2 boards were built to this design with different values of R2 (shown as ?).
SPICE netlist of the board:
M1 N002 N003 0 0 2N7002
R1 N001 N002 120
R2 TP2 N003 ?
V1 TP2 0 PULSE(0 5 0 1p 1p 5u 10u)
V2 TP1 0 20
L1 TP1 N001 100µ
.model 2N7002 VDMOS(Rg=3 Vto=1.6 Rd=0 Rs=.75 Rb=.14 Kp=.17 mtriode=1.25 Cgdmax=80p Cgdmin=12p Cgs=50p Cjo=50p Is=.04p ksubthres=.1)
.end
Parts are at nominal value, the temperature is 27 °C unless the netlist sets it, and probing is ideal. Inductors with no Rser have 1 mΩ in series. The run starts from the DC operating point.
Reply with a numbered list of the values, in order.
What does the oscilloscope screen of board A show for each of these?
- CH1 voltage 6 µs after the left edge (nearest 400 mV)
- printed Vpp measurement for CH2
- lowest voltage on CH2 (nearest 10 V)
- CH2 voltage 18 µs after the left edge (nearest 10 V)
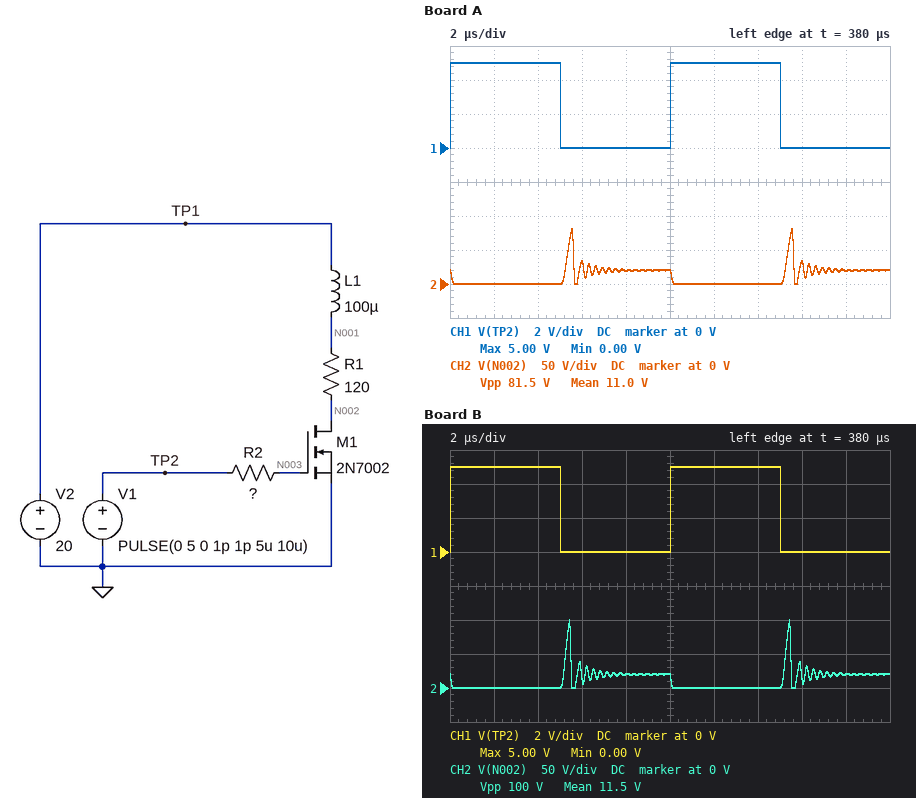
1. 0 V
2. 81.5 V
3. 0 V
4. 20 V
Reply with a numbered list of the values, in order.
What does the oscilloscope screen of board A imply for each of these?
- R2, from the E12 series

1. 1 kΩ
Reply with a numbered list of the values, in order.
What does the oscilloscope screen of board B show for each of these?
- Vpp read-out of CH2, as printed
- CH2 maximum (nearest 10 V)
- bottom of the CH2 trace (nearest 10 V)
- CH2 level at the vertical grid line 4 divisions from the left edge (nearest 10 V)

1. 100 V
2. 100 V
3. 0 V
4. 20 V
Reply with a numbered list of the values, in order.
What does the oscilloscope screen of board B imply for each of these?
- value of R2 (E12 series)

1. 680 Ω
